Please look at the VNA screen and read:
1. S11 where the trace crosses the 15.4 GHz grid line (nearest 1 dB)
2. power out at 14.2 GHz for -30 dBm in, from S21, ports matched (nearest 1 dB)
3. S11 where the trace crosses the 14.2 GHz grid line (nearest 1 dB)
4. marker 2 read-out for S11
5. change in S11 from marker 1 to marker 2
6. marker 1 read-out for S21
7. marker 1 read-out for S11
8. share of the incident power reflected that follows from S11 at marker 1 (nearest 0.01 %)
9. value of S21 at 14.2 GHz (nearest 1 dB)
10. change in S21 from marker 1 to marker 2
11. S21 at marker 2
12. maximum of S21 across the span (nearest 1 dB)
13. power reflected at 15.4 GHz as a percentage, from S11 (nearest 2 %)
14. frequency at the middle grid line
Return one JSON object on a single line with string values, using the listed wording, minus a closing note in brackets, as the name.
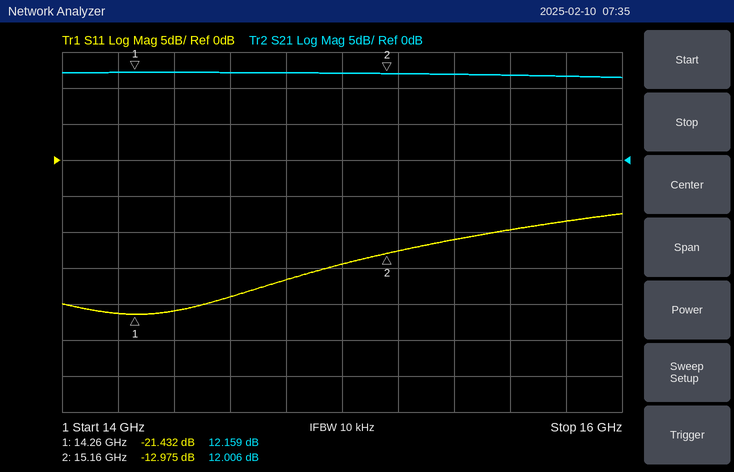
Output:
{"S11 where the trace crosses the 15.4 GHz grid line": "-11 dB", "power out at 14.2 GHz for -30 dBm in, from S21, ports matched": "-18 dBm", "S11 where the trace crosses the 14.2 GHz grid line": "-21 dB", "marker 2 read-out for S11": "-12.975 dB", "change in S11 from marker 1 to marker 2": "8.457 dB", "marker 1 read-out for S21": "12.159 dB", "marker 1 read-out for S11": "-21.432 dB", "share of the incident power reflected that follows from S11 at marker 1": "0.72 %", "value of S21 at 14.2 GHz": "12 dB", "change in S21 from marker 1 to marker 2": "-0.153 dB", "S21 at marker 2": "12.006 dB", "maximum of S21 across the span": "12 dB", "power reflected at 15.4 GHz as a percentage, from S11": "8 %", "frequency at the middle grid line": "15 GHz"}
